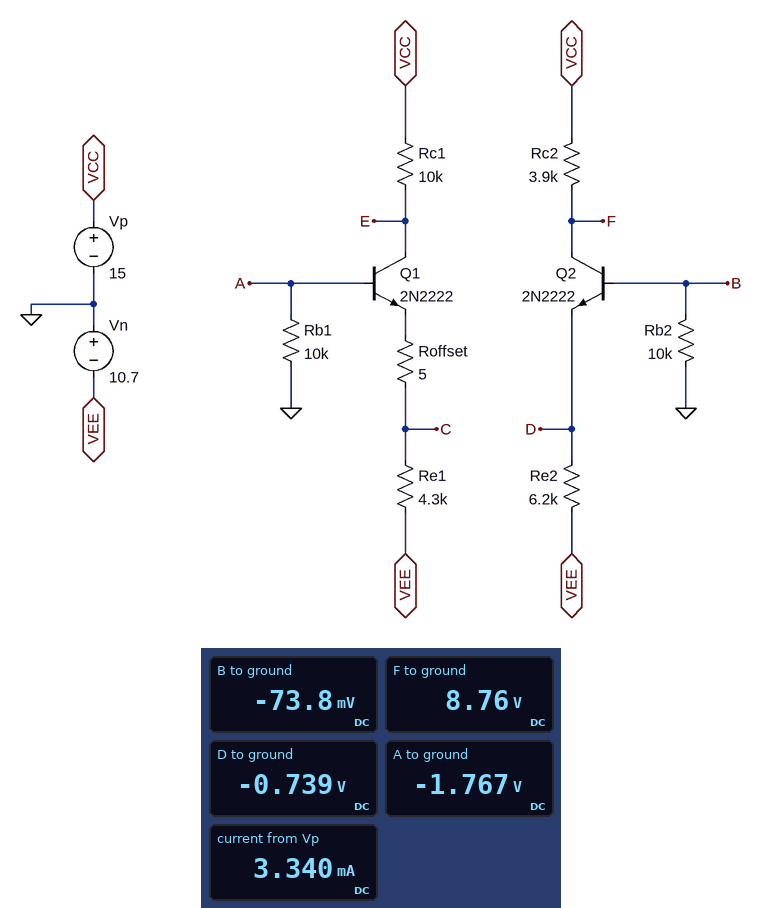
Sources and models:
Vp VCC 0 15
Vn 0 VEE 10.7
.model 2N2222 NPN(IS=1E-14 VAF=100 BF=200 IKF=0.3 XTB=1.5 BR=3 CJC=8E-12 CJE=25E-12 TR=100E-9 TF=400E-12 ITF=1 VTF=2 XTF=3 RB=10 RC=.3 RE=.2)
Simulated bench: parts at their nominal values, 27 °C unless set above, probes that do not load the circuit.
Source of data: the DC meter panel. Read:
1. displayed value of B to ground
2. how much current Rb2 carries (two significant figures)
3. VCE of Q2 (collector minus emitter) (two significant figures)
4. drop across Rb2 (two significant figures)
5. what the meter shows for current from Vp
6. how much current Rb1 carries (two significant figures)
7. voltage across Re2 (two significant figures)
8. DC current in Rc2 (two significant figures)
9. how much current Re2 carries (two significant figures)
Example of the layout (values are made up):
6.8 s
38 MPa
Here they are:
-73.8 mV
7.4 µA
9.5 V
74 mV
3.340 mA
180 µA
10 V
1.6 mA
1.6 mA
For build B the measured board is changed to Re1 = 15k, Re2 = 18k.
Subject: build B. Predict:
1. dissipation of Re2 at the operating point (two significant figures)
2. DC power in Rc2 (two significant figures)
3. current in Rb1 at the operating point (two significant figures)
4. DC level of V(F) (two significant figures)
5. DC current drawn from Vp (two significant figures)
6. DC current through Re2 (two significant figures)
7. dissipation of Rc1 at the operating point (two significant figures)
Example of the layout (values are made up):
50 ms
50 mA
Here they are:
5.6 mW
1.2 mW
3.1 µA
13 V
1.2 mA
560 µA
4.4 mW
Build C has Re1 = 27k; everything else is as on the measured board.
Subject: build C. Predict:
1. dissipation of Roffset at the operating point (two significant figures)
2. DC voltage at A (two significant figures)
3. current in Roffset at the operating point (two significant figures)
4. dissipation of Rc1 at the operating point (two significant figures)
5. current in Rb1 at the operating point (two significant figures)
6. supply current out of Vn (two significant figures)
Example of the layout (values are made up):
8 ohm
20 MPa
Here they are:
690 nW
-17 mV
370 µA
1.4 mW
1.7 µA
2.0 mA
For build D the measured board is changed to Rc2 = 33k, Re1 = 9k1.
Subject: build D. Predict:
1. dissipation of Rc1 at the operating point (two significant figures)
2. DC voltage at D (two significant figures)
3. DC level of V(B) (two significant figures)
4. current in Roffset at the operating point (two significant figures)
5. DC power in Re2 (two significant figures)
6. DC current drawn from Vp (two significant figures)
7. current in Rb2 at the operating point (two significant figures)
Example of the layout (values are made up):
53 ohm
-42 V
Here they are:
12 mW
-4.6 V
-3.9 V
1.1 mA
6.0 mW
1.7 mA
390 µA
